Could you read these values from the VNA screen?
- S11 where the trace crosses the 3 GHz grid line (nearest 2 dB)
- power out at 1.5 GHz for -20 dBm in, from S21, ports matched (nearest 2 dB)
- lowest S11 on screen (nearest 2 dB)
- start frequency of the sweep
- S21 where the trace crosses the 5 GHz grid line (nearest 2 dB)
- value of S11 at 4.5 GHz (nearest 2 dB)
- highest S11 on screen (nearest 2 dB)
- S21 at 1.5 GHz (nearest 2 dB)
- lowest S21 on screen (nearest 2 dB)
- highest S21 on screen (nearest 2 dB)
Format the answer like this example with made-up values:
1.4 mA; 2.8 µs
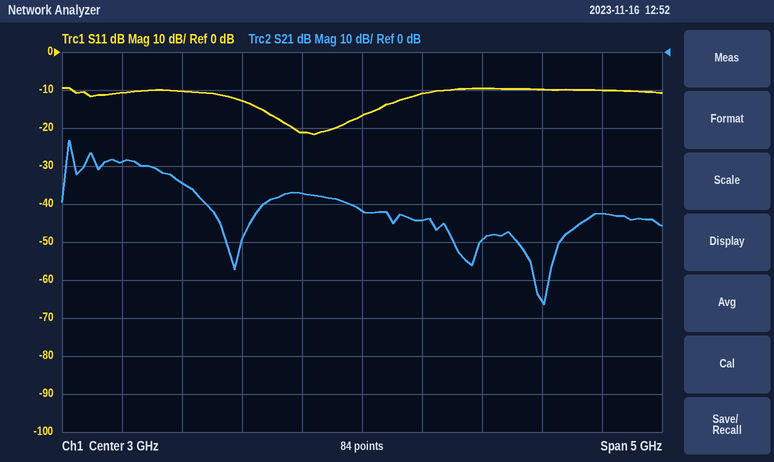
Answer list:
-16 dB; -54 dBm; -22 dB; 500 MHz; -42 dB; -10 dB; -10 dB; -34 dB; -66 dB; -24 dB
